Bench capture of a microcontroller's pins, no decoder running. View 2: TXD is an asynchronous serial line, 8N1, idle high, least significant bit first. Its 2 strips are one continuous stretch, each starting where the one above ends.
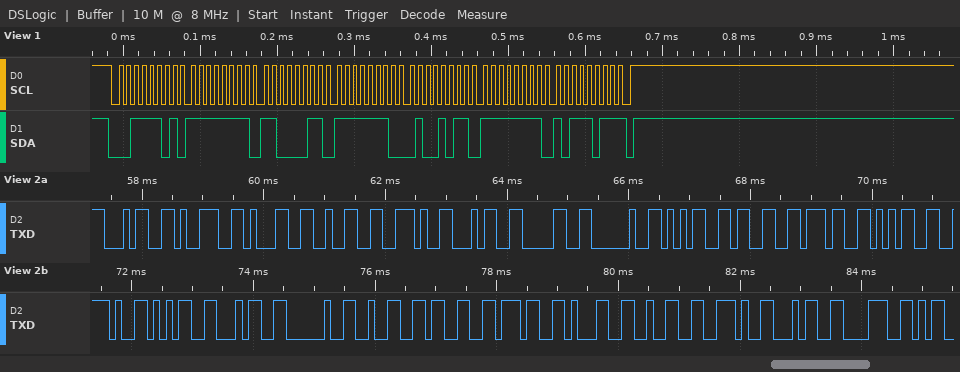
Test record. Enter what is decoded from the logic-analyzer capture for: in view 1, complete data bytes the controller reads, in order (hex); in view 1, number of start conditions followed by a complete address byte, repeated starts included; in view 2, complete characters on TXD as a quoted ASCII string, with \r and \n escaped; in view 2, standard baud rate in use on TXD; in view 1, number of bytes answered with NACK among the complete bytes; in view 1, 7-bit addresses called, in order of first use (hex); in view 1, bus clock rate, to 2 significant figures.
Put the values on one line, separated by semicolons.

FF C3 FE 4B FF BB; 1; "4912.40 5375.54 23712.48"; 9600 baud; 1; 0x1E; 100 kHz
